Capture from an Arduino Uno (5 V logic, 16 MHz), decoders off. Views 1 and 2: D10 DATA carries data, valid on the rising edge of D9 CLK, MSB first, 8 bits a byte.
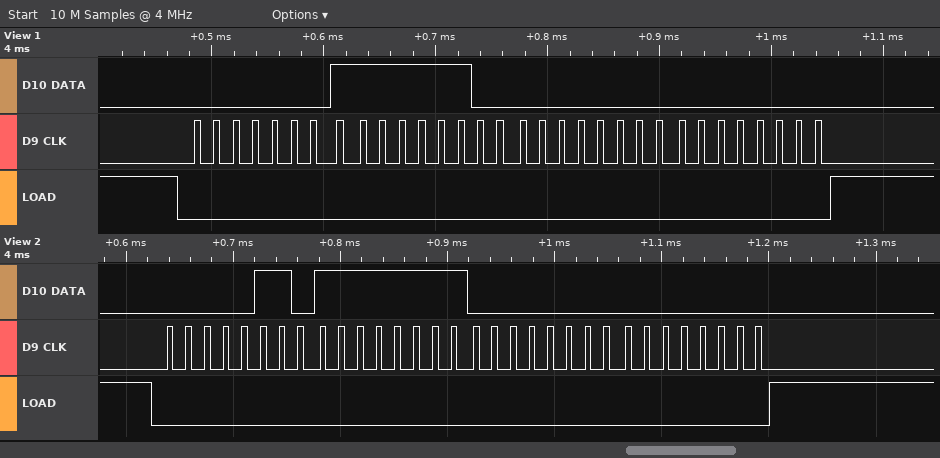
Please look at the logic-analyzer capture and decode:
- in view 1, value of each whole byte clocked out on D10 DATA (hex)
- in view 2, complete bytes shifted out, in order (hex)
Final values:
01 FC 00 00
06 FF 00 00
